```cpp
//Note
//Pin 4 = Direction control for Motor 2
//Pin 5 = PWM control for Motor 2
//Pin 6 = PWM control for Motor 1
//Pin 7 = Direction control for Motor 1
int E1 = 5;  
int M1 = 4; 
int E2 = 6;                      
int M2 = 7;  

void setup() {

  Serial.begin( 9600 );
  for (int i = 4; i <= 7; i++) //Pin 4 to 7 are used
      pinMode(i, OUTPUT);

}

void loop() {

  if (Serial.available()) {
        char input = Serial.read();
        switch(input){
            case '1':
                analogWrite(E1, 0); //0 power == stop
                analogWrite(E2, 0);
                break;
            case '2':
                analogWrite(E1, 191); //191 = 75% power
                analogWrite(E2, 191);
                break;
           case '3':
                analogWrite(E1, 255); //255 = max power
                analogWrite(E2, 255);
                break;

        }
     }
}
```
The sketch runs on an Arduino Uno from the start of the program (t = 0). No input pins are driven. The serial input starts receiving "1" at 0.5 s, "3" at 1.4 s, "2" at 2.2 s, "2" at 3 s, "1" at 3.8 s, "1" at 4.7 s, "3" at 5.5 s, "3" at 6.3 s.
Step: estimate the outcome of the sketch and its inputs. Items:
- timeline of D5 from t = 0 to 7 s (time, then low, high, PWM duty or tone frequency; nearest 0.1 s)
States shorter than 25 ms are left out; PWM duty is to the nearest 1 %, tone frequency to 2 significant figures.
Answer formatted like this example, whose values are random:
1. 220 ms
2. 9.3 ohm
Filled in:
1. 0 s low; 1.4 s high; 2.2 s PWM 75 %; 3.8 s low; 5.5 s high
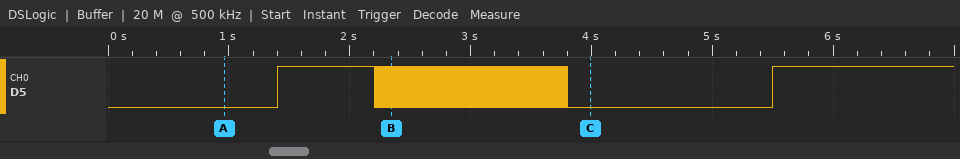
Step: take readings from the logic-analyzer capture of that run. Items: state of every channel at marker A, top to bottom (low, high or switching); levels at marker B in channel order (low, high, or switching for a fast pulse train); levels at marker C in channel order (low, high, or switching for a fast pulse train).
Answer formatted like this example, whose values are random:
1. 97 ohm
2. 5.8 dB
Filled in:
1. D5 low
2. D5 switching
3. D5 low
